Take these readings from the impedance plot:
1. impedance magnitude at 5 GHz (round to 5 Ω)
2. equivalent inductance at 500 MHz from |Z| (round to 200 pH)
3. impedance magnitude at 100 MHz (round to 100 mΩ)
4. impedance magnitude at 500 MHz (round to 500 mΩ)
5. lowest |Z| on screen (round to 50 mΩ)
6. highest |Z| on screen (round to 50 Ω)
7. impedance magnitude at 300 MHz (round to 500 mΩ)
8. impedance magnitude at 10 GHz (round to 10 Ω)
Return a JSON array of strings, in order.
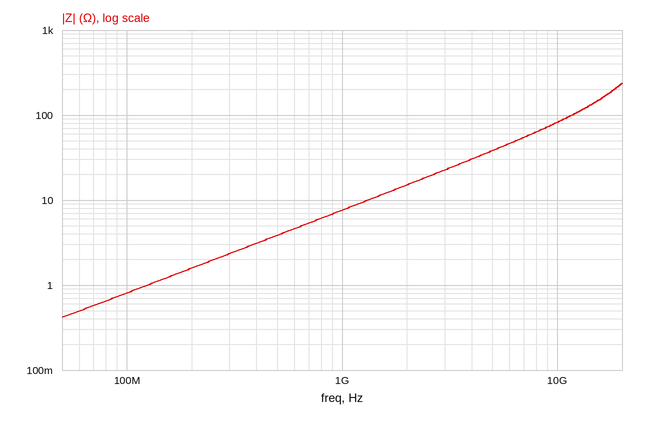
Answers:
["40 Ω", "1.2 nH", "800 mΩ", "4.0 Ω", "400 mΩ", "250 Ω", "2.5 Ω", "80 Ω"]
